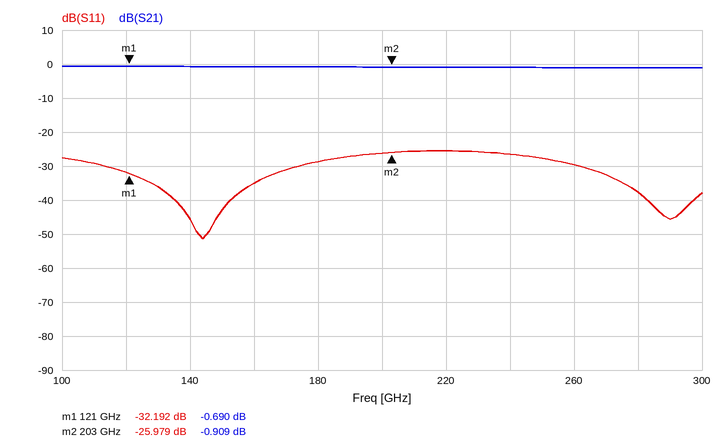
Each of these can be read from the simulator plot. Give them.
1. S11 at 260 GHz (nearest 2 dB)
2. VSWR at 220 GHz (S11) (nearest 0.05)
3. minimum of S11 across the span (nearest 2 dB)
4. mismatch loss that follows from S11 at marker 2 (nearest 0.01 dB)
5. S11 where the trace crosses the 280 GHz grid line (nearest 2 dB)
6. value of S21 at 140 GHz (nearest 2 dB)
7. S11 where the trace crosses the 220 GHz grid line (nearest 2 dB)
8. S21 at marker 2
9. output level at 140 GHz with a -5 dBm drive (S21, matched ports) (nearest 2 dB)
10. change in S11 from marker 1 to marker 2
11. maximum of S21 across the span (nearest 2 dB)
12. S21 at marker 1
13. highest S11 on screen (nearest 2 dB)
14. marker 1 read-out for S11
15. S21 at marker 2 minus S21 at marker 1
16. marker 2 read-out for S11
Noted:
-30 dB
1.10
-52 dB
0.01 dB
-38 dB
0 dB
-26 dB
-0.909 dB
-6 dBm
6.213 dB
0 dB
-0.690 dB
-26 dB
-32.192 dB
-0.219 dB
-25.979 dB
